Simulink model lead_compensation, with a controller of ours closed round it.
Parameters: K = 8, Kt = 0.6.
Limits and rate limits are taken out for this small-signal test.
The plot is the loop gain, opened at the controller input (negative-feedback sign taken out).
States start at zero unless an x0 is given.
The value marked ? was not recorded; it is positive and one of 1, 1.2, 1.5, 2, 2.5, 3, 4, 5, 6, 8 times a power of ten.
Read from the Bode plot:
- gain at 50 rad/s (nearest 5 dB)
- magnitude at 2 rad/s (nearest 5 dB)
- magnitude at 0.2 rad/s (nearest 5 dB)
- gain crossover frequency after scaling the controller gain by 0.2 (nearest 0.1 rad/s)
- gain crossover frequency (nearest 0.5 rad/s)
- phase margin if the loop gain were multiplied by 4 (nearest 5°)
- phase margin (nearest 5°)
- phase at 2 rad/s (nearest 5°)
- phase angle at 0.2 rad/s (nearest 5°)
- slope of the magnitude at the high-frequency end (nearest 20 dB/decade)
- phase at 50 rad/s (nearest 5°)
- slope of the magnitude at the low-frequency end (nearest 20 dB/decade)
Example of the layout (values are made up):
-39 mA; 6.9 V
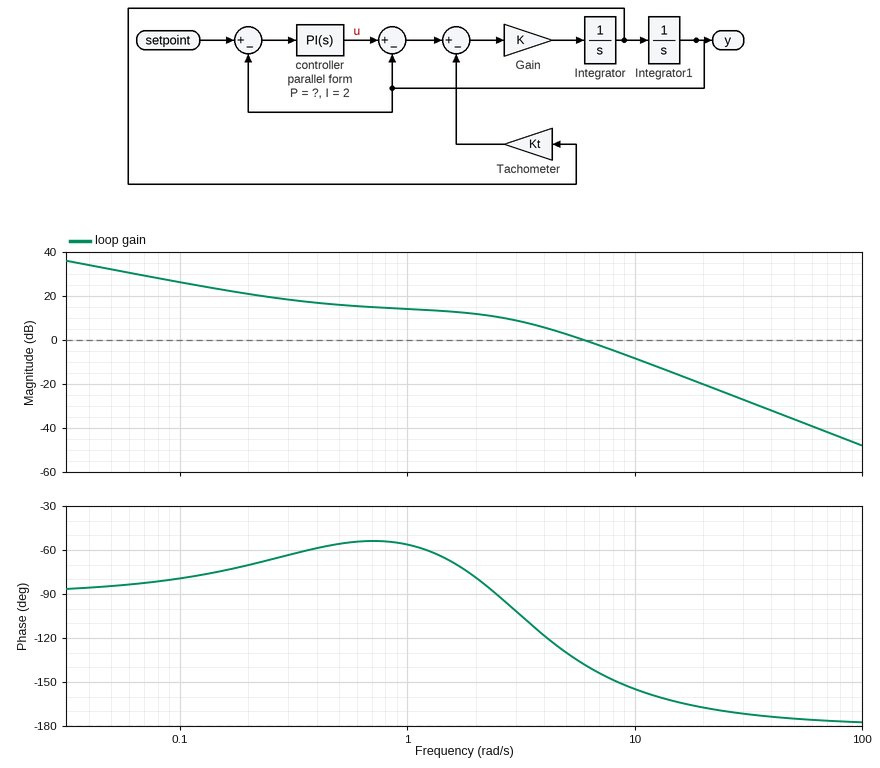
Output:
-35 dB; 10 dB; 20 dB; 1.1 rad/s; 6.0 rad/s; 20°; 40°; -80°; -70°; -40 dB/decade; -175°; -20 dB/decade
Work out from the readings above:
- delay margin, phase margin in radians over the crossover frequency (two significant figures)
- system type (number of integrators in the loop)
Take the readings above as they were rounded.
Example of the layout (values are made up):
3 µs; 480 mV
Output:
0.12 s; 1
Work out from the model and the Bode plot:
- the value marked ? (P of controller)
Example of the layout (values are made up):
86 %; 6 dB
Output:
5
